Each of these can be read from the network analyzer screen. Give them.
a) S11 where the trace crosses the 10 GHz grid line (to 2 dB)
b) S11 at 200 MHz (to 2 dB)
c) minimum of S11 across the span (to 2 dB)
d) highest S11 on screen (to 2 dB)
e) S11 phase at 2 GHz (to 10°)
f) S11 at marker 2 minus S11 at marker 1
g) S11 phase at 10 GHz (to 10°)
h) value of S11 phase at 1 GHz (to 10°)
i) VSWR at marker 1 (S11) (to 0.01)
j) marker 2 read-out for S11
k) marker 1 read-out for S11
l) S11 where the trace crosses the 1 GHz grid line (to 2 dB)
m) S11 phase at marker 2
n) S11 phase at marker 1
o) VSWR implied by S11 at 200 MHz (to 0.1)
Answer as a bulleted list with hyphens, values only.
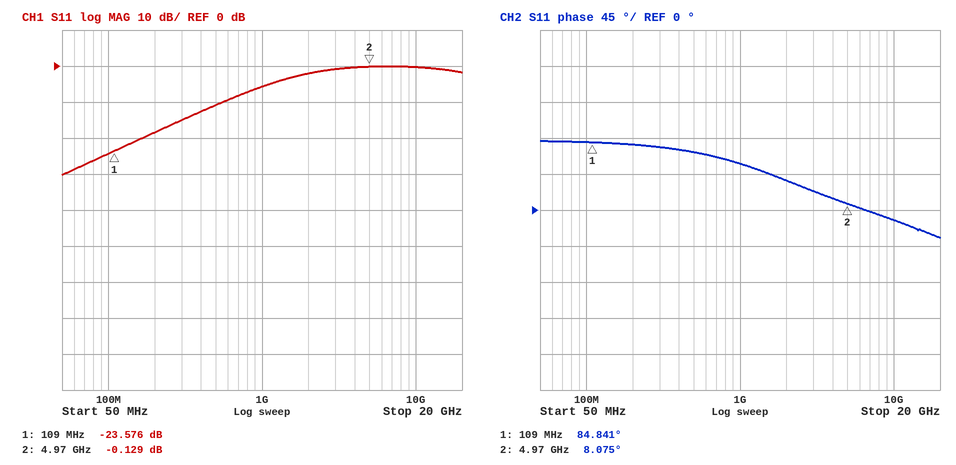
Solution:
- 0 dB
- -18 dB
- -30 dB
- 0 dB
- 40°
- 23.447 dB
- -10°
- 60°
- 1.14
- -0.129 dB
- -23.576 dB
- -6 dB
- 8.075°
- 84.841°
- 1.3
